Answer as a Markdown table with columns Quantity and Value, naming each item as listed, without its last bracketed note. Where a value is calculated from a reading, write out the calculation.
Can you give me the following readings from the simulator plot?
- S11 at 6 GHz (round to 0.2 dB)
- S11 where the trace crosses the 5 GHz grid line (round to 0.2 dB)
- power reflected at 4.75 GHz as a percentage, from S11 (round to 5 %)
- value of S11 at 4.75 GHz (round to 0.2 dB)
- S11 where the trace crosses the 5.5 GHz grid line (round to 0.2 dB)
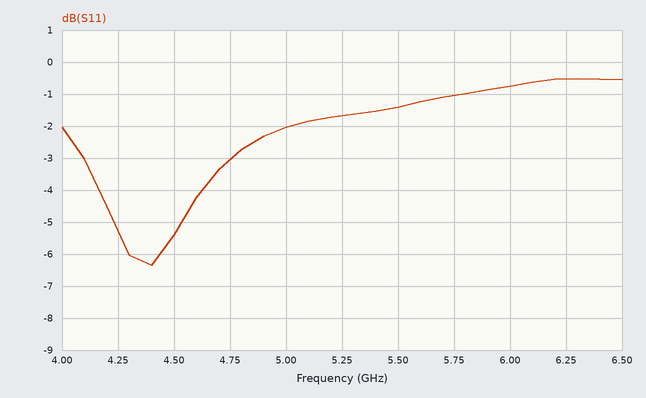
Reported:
| Quantity | Value |
|---|---|
| S11 at 6 GHz | -0.8 dB |
| S11 where the trace crosses the 5 GHz grid line | -2.0 dB |
| power reflected at 4.75 GHz as a percentage, from S11 | 10^(-3/10) ≈ 50 % |
| value of S11 at 4.75 GHz | -3.0 dB |
| S11 where the trace crosses the 5.5 GHz grid line | -1.4 dB |
